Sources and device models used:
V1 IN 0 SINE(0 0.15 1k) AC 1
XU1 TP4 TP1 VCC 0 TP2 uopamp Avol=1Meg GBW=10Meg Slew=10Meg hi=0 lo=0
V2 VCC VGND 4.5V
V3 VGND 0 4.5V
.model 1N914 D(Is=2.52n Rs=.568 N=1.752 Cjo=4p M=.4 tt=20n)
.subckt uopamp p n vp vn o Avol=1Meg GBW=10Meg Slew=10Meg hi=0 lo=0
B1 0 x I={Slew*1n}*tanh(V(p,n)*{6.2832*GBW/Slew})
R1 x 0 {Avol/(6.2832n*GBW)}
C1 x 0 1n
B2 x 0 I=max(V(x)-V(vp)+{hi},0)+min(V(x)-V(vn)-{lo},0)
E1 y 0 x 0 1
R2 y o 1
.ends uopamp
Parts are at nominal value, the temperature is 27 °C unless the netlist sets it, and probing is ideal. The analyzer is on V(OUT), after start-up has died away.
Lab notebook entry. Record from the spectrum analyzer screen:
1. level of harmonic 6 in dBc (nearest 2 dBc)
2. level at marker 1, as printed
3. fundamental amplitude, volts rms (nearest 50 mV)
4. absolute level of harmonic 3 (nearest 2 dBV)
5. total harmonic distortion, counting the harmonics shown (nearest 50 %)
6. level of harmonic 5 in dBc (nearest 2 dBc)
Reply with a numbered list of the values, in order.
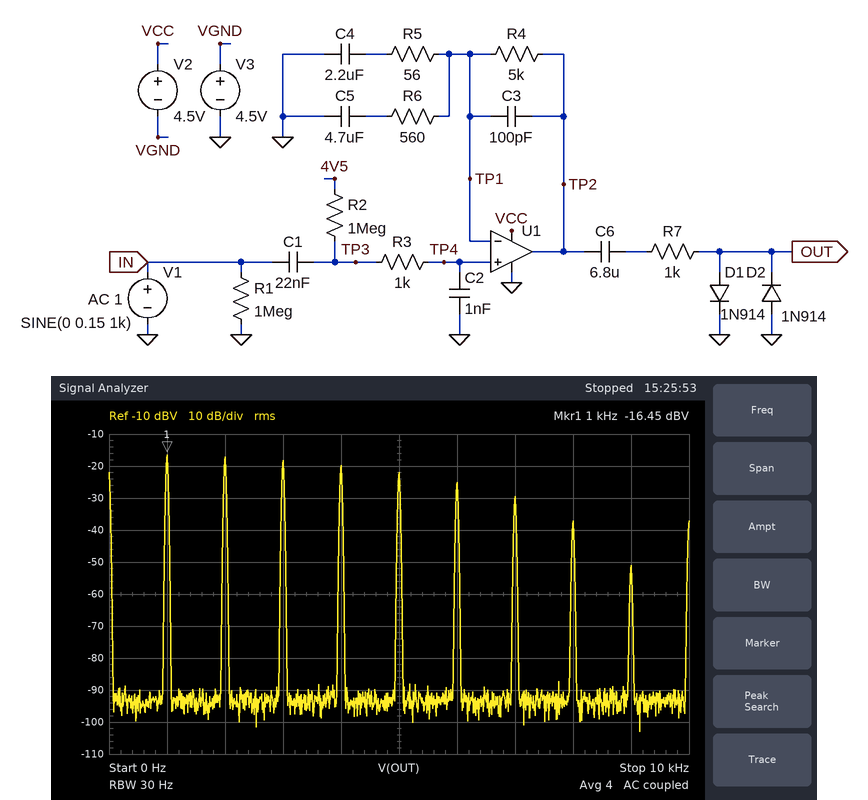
1. -8 dBc
2. -16.45 dBV
3. 150 mV
4. -18 dBV
5. 150 %
6. -6 dBc
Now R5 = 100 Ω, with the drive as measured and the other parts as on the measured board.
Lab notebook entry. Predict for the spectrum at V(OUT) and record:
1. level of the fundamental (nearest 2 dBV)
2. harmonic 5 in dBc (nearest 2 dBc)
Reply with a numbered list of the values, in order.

1. -16 dBV
2. -8 dBc
